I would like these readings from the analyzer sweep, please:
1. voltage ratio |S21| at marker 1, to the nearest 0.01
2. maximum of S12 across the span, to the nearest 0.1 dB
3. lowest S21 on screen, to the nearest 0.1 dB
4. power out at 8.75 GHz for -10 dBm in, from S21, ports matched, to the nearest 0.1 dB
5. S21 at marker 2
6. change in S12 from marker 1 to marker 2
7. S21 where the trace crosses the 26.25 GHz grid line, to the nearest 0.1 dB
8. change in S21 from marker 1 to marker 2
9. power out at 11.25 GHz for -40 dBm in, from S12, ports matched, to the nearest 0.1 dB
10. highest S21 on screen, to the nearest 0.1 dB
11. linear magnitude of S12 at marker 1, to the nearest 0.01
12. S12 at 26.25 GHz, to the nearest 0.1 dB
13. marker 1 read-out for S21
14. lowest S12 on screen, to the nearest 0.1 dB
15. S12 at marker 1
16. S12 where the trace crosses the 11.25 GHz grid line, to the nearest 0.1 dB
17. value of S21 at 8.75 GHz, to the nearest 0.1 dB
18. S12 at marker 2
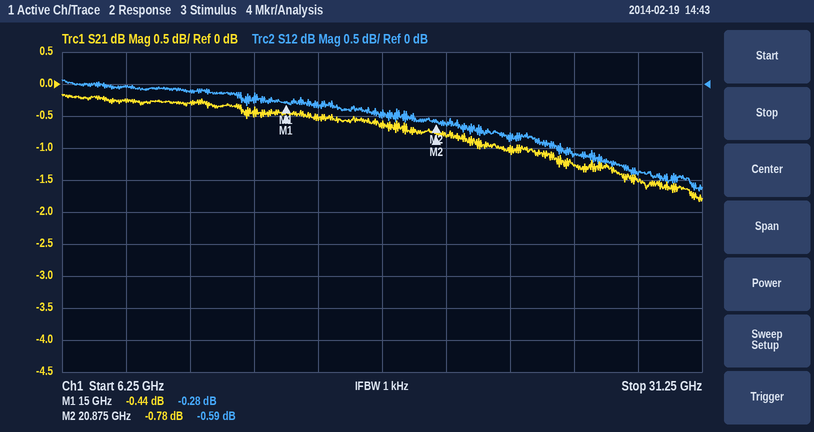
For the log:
0.95
0.1 dB
-1.8 dB
-10.3 dBm
-0.78 dB
-0.31 dB
-1.3 dB
-0.34 dB
-40.1 dBm
-0.2 dB
0.97
-1.1 dB
-0.44 dB
-1.7 dB
-0.28 dB
-0.1 dB
-0.3 dB
-0.59 dB
